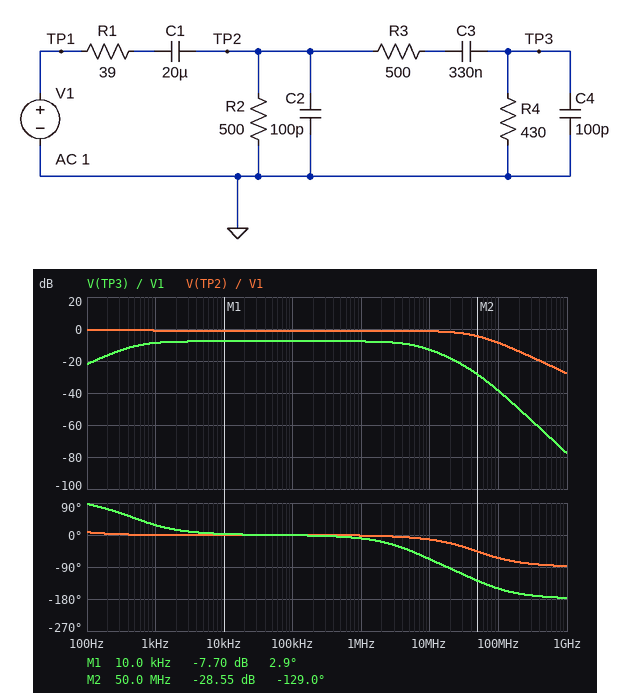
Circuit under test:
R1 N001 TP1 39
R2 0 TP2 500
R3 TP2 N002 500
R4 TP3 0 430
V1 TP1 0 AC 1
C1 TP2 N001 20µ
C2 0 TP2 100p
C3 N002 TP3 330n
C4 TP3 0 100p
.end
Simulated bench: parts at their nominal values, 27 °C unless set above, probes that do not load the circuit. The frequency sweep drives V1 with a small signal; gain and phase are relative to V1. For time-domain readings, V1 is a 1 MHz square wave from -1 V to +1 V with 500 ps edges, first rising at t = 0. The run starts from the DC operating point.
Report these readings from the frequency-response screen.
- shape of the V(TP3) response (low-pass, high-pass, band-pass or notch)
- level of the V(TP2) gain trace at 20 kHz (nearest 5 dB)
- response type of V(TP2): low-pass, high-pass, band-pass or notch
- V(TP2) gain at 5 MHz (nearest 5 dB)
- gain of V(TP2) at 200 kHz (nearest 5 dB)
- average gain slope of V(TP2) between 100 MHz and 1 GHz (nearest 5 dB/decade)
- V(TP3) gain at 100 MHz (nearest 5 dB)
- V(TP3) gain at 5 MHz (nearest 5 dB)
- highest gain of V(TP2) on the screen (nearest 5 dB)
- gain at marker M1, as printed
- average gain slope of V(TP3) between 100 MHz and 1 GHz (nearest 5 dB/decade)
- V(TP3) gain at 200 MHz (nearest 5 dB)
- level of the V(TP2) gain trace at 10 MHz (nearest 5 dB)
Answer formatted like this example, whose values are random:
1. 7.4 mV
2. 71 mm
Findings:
1. band-pass
2. 0 dB
3. low-pass
4. 0 dB
5. 0 dB
6. -20 dB/decade
7. -40 dB
8. -10 dB
9. 0 dB
10. -7.70 dB
11. -40 dB/decade
12. -50 dB
13. 0 dB
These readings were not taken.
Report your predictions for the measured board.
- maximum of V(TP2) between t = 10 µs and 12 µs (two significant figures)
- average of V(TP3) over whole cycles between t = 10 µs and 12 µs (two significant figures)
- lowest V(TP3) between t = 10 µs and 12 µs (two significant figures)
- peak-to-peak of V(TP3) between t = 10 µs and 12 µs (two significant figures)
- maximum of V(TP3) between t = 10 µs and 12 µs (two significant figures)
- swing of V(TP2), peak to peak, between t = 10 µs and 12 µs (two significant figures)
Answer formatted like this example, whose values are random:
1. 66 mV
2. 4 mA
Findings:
1. 1.8 V
2. 400 mV
3. -16 mV
4. 830 mV
5. 810 mV
6. 1.8 V
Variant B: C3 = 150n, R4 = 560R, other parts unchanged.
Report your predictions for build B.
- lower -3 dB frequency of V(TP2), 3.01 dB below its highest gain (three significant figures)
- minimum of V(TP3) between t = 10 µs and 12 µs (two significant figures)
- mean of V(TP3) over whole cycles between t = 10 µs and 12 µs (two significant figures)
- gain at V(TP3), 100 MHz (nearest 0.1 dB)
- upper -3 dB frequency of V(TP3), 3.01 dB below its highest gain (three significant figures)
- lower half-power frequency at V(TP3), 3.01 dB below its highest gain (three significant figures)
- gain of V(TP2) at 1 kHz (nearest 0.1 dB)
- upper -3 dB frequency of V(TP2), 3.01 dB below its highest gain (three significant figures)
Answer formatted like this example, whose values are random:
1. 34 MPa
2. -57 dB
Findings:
1. 14.6 Hz
2. -34 mV
3. 440 mV
4. -38.6 dB
5. 5.70 MHz
6. 974 Hz
7. -0.8 dB
8. 41.3 MHz
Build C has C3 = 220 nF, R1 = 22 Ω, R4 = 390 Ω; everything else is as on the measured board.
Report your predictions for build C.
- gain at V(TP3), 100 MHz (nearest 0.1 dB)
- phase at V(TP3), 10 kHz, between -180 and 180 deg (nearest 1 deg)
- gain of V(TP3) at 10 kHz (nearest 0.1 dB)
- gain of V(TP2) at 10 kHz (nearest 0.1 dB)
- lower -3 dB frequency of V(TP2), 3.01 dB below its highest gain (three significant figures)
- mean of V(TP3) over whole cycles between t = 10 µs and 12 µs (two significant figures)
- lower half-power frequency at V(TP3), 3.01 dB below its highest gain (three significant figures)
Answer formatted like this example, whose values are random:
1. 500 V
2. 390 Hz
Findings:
1. -34.9 dB
2. 5 deg
3. -7.8 dB
4. -0.6 dB
5. 15.0 Hz
6. 390 mV
7. 802 Hz
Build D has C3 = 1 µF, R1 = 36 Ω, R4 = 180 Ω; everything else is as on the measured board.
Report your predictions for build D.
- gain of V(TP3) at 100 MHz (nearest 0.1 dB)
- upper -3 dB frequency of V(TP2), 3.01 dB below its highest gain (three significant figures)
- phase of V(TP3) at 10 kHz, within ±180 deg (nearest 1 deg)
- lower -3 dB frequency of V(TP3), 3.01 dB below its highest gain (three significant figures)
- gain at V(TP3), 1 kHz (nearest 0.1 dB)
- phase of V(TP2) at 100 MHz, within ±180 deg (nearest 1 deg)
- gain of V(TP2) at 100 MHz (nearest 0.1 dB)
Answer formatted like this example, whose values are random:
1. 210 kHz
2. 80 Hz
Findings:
1. -38.1 dB
2. 48.7 MHz
3. 1 deg
4. 234 Hz
5. -12.8 dB
6. -63 deg
7. -8.1 dB
